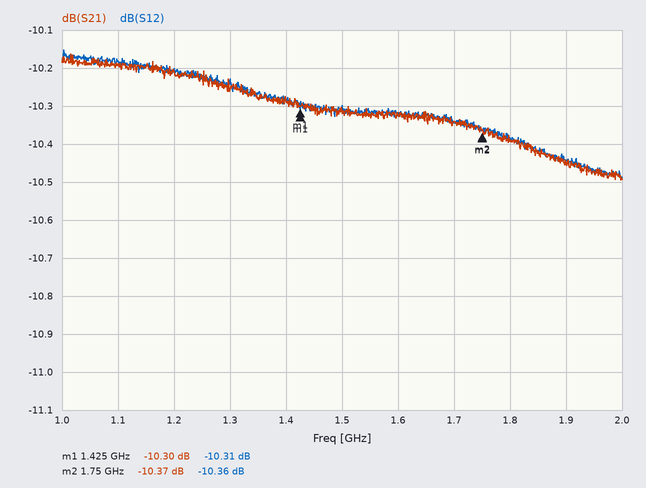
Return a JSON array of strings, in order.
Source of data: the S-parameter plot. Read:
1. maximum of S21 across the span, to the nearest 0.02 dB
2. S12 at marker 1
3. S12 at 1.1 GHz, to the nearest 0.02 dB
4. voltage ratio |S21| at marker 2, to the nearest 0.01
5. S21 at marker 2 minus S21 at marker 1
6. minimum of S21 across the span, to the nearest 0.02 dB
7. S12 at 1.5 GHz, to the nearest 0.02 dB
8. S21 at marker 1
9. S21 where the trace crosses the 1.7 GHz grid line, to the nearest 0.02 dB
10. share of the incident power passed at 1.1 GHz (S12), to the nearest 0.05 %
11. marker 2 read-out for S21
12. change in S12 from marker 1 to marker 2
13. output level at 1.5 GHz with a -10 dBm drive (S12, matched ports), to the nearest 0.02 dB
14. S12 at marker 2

["-10.16 dB", "-10.31 dB", "-10.18 dB", "0.30", "-0.07 dB", "-10.50 dB", "-10.30 dB", "-10.30 dB", "-10.34 dB", "9.60 %", "-10.37 dB", "-0.05 dB", "-20.30 dBm", "-10.36 dB"]
